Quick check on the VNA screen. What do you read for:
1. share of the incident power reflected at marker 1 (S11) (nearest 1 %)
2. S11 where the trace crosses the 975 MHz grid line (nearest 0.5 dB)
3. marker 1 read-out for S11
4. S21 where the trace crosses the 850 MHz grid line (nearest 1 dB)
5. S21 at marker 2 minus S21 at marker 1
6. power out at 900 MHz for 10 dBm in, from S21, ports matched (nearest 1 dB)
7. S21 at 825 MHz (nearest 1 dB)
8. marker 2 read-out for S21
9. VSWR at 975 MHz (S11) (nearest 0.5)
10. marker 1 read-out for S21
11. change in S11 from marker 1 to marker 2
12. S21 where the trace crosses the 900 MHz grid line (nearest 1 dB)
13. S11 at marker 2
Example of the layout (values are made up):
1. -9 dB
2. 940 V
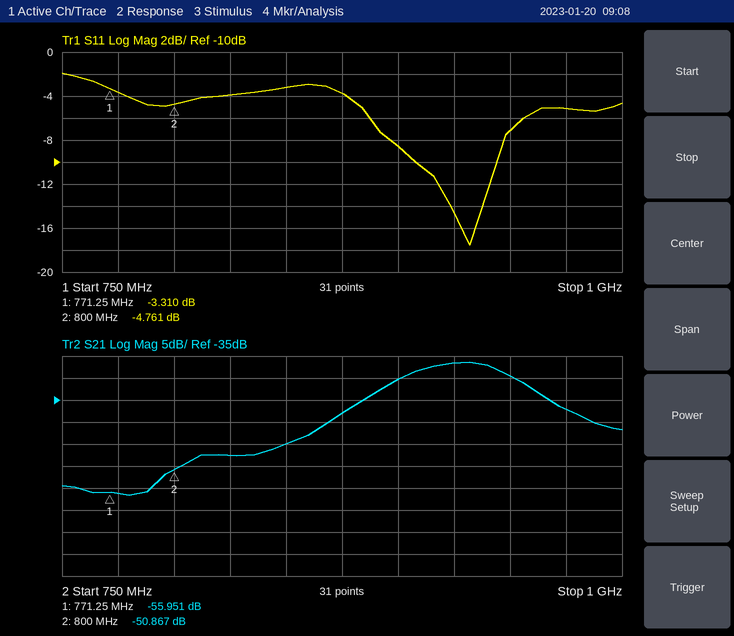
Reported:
1. 47 %
2. -5.0 dB
3. -3.310 dB
4. -45 dB
5. 5.084 dB
6. -20 dBm
7. -48 dB
8. -50.867 dB
9. 3.5
10. -55.951 dB
11. -1.451 dB
12. -30 dB
13. -4.761 dB
